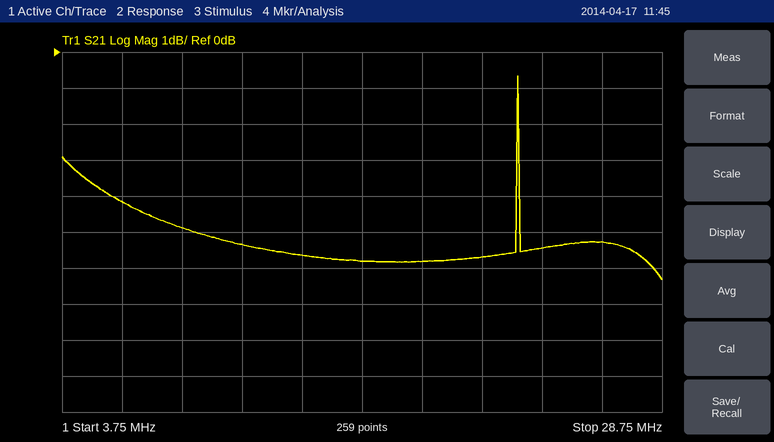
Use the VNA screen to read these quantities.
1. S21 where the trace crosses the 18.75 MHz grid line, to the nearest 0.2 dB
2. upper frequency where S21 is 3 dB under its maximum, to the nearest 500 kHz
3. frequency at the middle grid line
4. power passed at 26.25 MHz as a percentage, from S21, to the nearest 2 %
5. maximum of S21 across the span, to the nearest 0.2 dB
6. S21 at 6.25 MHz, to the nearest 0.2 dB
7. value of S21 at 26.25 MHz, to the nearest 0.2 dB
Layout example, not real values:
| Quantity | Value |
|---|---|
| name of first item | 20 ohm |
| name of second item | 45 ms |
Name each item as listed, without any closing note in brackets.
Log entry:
| Quantity | Value |
|---|---|
| S21 where the trace crosses the 18.75 MHz grid line, to the nearest 0.2 dB | -5.8 dB |
| upper frequency where S21 is 3 dB under its maximum, to the nearest 500 kHz | 23.0 MHz |
| frequency at the middle grid line | 16.25 MHz |
| power passed at 26.25 MHz as a percentage, from S21, to the nearest 2 % | 30 % |
| maximum of S21 across the span, to the nearest 0.2 dB | -0.6 dB |
| S21 at 6.25 MHz, to the nearest 0.2 dB | -4.2 dB |
| value of S21 at 26.25 MHz, to the nearest 0.2 dB | -5.2 dB |
